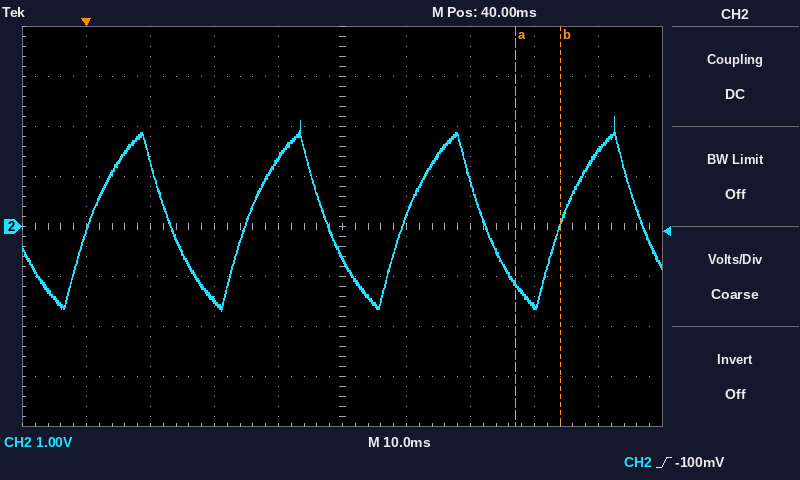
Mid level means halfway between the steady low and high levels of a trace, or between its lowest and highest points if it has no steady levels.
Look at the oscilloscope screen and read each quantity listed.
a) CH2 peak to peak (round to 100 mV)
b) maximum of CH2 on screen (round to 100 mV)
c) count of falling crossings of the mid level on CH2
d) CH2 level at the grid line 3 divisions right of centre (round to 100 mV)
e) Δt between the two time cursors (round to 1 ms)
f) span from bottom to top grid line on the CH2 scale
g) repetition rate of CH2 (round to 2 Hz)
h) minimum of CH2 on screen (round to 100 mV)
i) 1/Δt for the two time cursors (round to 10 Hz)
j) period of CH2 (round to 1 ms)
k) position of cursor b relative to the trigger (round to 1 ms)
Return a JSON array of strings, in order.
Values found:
["3.9 V", "2.2 V", "4", "-1.6 V", "7 ms", "8 V", "40 Hz", "-1.7 V", "140 Hz", "25 ms", "+74 ms"]
